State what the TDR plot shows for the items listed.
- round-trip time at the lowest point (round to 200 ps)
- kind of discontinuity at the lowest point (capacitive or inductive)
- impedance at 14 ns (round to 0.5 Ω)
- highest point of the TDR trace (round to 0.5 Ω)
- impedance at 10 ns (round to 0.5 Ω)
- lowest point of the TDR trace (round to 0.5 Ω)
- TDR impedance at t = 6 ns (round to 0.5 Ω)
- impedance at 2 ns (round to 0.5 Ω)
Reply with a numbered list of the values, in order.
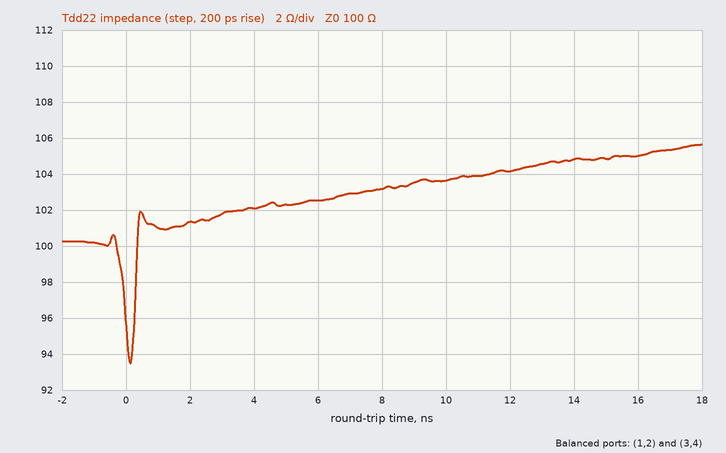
1. 200 ps
2. capacitive
3. 105.0 Ω
4. 105.5 Ω
5. 103.5 Ω
6. 93.5 Ω
7. 102.5 Ω
8. 101.5 Ω
